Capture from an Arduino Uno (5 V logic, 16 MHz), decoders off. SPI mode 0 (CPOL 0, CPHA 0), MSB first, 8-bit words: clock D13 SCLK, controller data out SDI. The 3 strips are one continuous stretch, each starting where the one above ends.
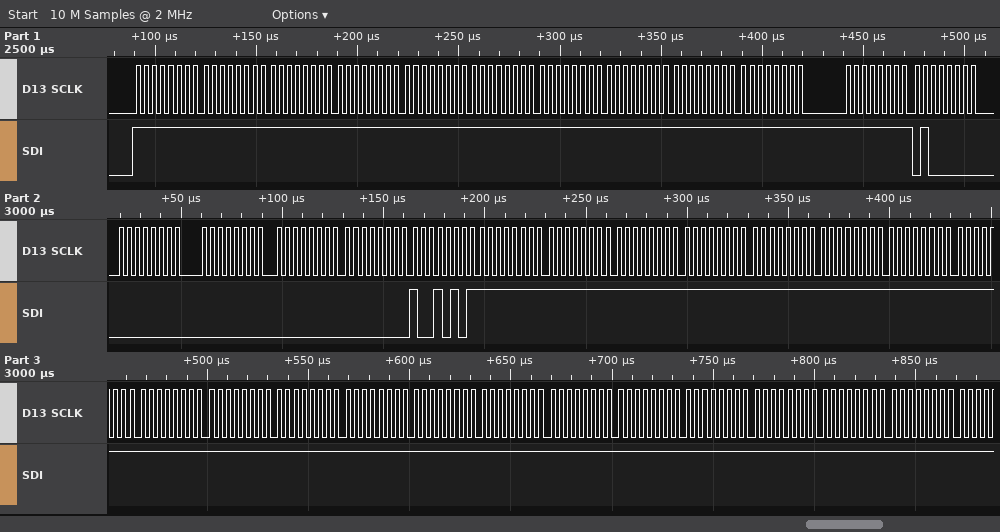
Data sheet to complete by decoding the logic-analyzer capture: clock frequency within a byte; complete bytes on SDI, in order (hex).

250 kHz
FF FF FF FF FF FF FF FF FF FF FF 40 00 00 00 00 95 FF FF FF FF FF FF FF FF FF FF FF FF FF FF FF FF FF FF FF FF
